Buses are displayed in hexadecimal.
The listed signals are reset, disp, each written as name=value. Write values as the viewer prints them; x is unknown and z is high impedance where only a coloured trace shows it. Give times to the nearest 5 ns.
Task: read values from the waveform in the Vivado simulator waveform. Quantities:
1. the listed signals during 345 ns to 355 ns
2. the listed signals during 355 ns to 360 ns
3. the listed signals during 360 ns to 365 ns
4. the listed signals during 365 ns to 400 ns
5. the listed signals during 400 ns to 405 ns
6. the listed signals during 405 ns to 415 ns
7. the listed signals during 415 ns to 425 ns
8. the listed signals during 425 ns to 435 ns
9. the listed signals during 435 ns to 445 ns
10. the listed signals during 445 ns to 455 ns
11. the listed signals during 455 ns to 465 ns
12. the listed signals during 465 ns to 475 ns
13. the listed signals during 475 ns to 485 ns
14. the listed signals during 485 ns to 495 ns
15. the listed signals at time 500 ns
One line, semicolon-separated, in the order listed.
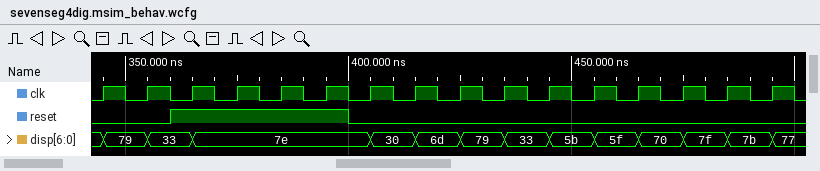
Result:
reset=0, disp=79; reset=0, disp=33; reset=1, disp=33; reset=1, disp=7e; reset=0, disp=7e; reset=0, disp=30; reset=0, disp=6d; reset=0, disp=79; reset=0, disp=33; reset=0, disp=5b; reset=0, disp=5f; reset=0, disp=70; reset=0, disp=7f; reset=0, disp=7b; reset=0, disp=77
